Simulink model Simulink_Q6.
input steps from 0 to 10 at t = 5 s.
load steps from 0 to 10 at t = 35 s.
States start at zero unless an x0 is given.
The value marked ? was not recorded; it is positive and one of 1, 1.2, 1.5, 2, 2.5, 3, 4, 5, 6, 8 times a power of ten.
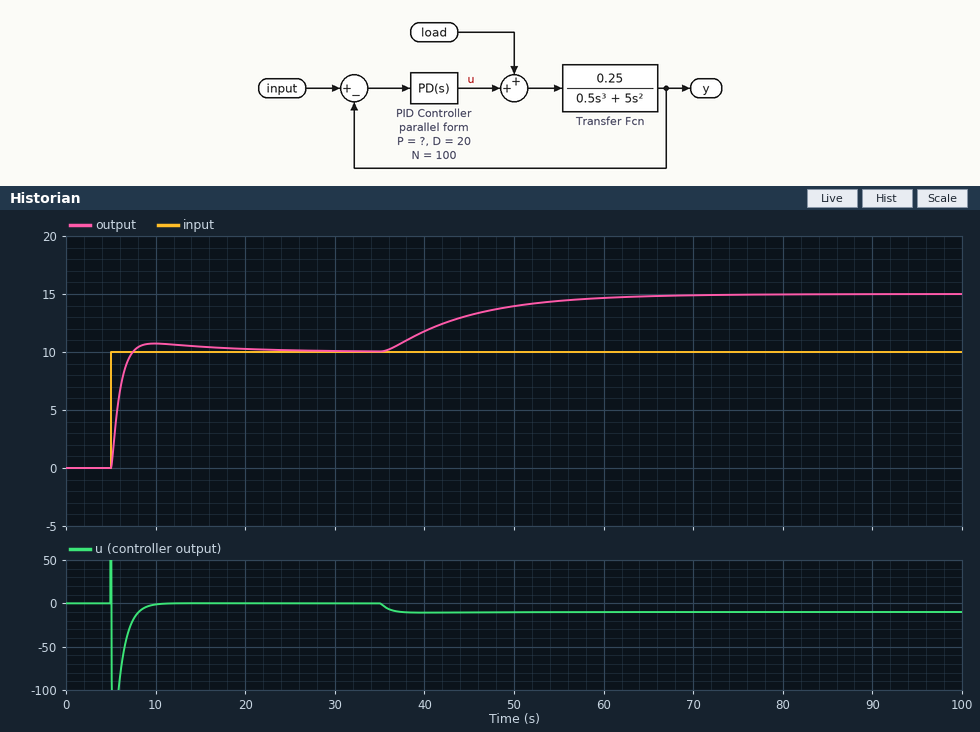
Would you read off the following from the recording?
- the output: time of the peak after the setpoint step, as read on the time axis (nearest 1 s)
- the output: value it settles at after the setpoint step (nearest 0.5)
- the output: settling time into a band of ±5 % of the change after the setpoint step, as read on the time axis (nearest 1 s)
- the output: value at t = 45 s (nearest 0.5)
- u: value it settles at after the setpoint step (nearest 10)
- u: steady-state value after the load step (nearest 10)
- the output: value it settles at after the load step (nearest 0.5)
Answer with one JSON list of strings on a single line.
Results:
["10 s", "10.0", "14 s", "13.0", "0", "-10", "15.0"]
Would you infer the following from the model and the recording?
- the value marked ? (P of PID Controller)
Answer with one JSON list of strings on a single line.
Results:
["2"]
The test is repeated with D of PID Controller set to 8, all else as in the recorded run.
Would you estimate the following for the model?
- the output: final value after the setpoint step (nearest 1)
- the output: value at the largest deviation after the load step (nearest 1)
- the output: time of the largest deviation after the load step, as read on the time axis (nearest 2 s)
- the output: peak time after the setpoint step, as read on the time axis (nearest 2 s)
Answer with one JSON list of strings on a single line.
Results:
["10", "15", "48 s", "12 s"]
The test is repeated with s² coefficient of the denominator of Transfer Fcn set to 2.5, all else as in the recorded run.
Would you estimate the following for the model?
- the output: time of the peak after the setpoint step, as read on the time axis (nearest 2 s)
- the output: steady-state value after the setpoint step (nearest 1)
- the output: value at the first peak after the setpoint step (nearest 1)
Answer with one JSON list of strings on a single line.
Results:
["6 s", "10", "11"]
